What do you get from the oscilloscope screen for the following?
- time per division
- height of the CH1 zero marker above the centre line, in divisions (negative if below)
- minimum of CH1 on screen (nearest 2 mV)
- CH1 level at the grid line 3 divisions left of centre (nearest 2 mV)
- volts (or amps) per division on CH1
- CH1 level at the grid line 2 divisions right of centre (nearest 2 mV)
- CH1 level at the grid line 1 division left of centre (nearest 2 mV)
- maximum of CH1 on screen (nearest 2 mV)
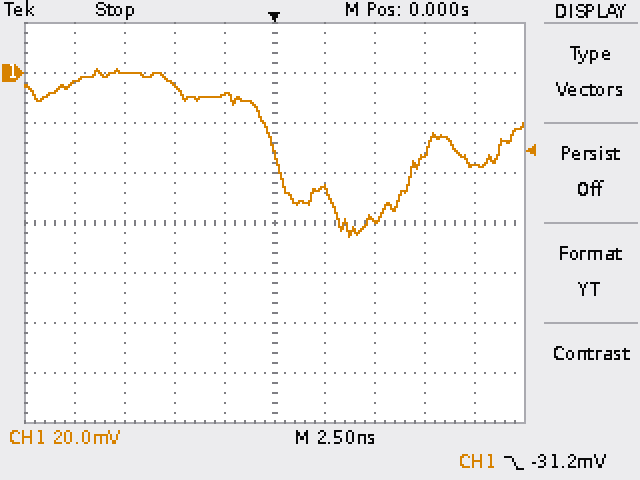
2.5 ns
+3.0 div
-66 mV
0 mV
20 mV
-58 mV
-8 mV
2 mV
